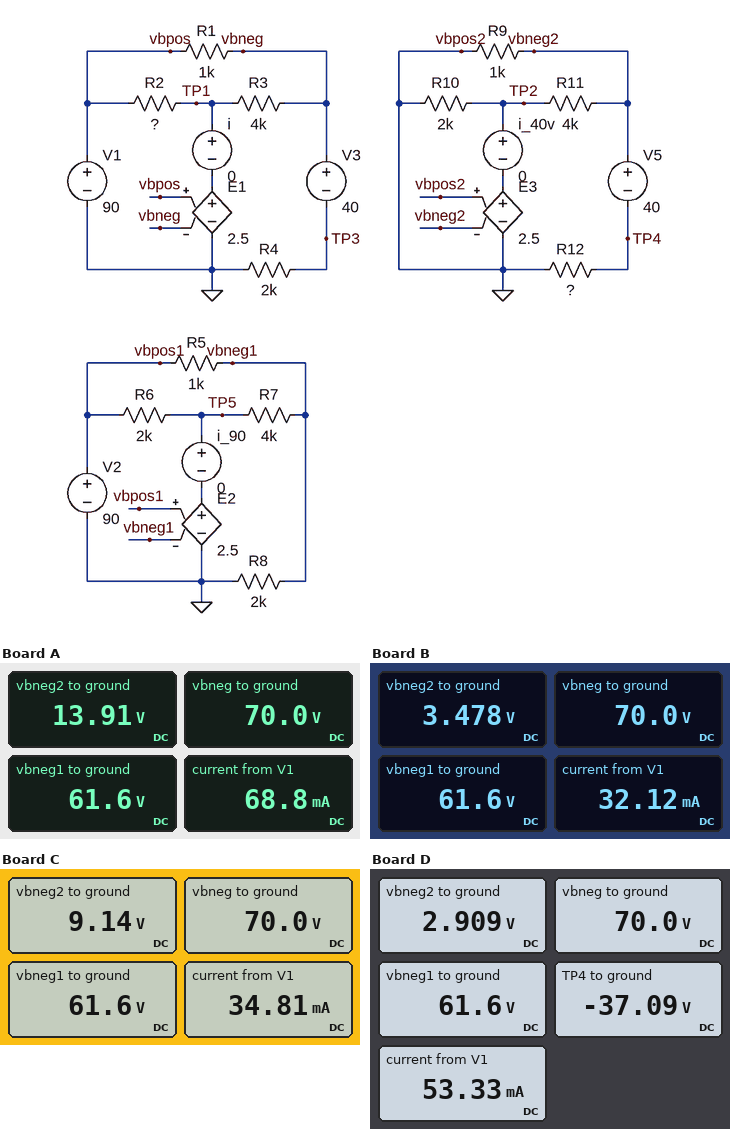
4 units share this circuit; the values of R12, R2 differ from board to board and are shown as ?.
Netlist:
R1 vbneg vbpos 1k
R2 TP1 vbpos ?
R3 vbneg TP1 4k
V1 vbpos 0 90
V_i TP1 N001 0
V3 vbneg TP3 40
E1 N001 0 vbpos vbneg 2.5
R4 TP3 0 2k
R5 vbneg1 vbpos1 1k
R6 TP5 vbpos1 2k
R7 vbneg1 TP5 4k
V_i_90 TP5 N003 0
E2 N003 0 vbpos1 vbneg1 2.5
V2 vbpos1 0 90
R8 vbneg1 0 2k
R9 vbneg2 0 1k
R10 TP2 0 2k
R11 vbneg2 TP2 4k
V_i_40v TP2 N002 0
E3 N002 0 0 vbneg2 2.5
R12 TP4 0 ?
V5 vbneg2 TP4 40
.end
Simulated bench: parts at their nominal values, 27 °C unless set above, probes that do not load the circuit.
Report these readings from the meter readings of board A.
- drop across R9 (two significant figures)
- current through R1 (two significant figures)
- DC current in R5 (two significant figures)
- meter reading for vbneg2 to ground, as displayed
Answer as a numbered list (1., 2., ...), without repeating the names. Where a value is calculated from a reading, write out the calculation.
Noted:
1. 13.91 V = 14 V
2. (90 V - 70 V) / 1 kΩ = 20 mA
3. (90 V - 61.6 V) / 1 kΩ = 28 mA
4. 13.91 V
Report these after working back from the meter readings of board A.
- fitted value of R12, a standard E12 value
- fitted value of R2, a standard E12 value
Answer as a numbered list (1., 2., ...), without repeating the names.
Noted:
1. 1 kΩ
2. 820 Ω
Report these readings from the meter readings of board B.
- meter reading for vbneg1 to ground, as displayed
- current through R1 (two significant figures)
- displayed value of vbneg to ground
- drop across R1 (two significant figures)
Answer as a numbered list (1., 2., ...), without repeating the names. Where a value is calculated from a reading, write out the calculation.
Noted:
1. 61.6 V
2. (90 V - 70 V) / 1 kΩ = 20 mA
3. 70.0 V
4. 90 V - 70 V = 20 V
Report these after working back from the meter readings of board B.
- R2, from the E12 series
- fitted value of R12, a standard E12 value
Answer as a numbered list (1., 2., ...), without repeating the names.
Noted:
1. 3.3 kΩ
2. 5.6 kΩ
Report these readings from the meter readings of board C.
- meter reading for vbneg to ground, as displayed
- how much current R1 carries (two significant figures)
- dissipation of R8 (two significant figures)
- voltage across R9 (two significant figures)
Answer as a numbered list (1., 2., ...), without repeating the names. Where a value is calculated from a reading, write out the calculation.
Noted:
1. 70.0 V
2. (90 V - 70 V) / 1 kΩ = 20 mA
3. (61.6 V)^2 / 2 kΩ = 1.9 W
4. 9.14 V = 9.1 V
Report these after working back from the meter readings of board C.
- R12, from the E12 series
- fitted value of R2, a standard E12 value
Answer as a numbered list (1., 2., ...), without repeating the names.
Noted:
1. 1.8 kΩ
2. 2.7 kΩ
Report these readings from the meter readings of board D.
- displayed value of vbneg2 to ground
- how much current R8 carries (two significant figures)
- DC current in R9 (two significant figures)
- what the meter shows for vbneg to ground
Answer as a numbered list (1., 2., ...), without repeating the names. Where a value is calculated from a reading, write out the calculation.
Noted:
1. 2.909 V
2. (61.6 V) / 2 kΩ = 31 mA
3. (2.909 V) / 1 kΩ = 2.9 mA
4. 70.0 V
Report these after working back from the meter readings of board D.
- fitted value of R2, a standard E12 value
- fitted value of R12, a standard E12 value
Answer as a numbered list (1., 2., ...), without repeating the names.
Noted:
1. 1.2 kΩ
2. 6.8 kΩ
